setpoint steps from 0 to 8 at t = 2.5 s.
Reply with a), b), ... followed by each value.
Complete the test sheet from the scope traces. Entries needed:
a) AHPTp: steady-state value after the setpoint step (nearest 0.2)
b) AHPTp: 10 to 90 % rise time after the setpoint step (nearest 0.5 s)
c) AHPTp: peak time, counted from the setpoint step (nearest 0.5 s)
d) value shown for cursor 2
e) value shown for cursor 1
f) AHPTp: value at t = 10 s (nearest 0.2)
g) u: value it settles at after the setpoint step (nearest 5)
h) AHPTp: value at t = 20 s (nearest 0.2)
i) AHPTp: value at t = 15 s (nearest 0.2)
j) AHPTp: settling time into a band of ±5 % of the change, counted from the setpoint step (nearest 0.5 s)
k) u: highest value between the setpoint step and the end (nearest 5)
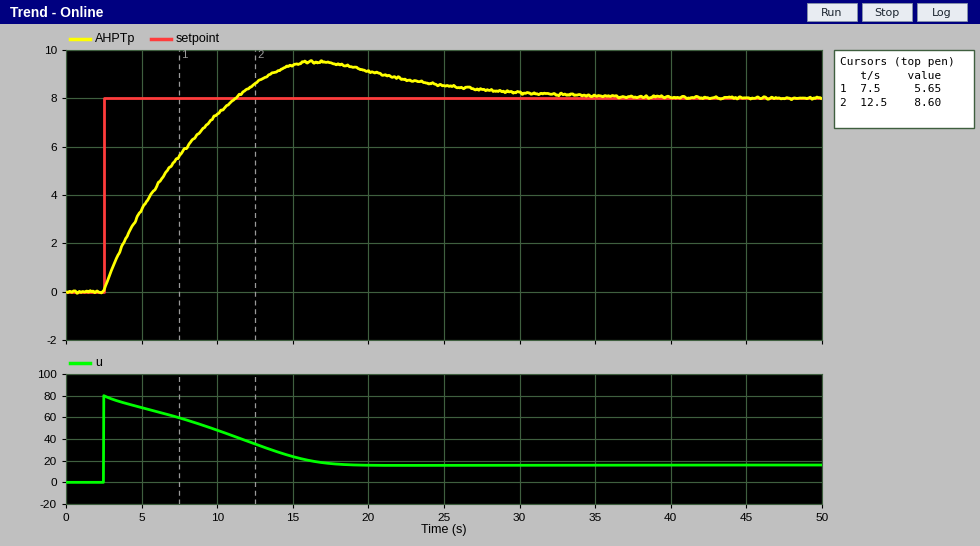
a) 8.0
b) 7.0 s
c) 14.0 s
d) 8.60
e) 5.65
f) 7.4
g) 15
h) 9.2
i) 9.4
j) 24.5 s
k) 80
